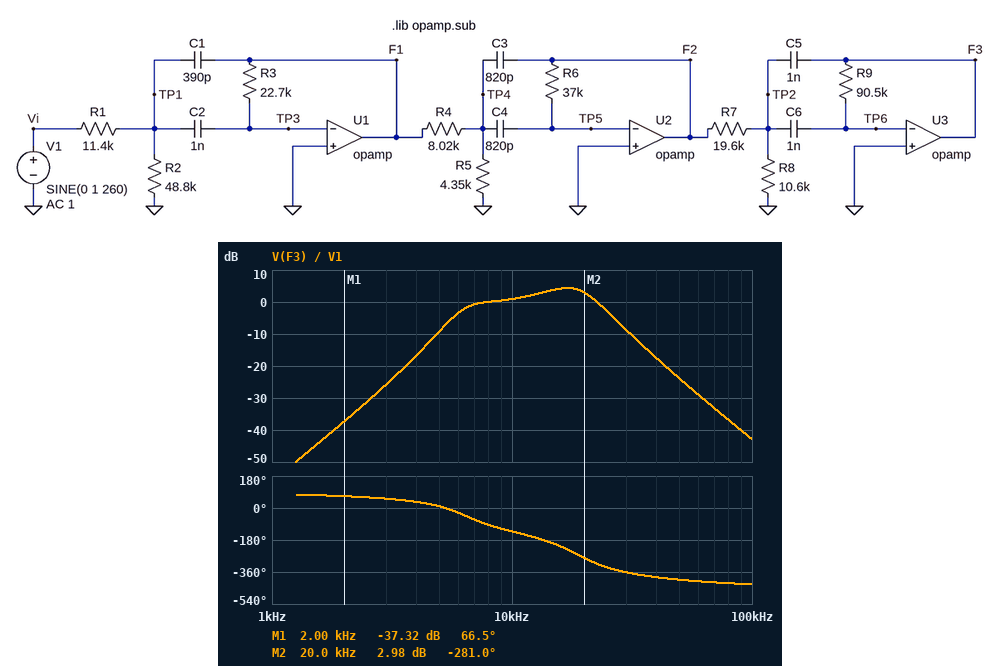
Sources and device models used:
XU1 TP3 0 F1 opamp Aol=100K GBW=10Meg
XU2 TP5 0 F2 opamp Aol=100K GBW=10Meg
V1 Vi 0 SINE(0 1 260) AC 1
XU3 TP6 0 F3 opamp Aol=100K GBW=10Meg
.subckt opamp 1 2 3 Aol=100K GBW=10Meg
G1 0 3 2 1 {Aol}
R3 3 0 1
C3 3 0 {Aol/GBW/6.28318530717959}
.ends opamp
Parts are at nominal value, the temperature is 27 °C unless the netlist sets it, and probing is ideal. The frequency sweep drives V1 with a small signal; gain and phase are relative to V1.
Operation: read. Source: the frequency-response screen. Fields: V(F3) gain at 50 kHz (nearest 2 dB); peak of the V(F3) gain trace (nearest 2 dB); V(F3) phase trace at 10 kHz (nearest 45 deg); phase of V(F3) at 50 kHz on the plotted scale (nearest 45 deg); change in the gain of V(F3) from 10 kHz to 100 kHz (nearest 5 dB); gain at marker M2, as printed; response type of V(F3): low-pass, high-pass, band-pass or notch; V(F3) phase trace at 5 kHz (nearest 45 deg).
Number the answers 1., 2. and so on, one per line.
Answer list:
1. -24 dB
2. 4 dB
3. -135 deg
4. -405 deg
5. -45 dB
6. 2.98 dB
7. band-pass
8. 0 deg
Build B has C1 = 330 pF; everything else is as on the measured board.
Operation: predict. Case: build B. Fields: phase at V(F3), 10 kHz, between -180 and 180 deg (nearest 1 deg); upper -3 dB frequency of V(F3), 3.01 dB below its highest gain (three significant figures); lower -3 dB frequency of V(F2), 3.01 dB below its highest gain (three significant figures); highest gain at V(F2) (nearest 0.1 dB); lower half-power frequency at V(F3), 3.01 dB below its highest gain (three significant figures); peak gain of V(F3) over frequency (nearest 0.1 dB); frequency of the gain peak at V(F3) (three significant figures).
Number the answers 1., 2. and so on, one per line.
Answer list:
1. -128 deg
2. 21.8 kHz
3. 14.9 kHz
4. 10.8 dB
5. 11.4 kHz
6. 4.7 dB
7. 17.3 kHz
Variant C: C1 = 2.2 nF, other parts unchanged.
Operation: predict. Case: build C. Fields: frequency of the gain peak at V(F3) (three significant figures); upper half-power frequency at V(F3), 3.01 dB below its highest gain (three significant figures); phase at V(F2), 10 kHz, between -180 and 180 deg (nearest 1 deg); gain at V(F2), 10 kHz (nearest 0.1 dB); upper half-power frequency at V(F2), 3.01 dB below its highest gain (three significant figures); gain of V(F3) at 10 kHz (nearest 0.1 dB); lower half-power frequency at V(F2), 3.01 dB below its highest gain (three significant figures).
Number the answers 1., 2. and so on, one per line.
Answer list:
1. 7.17 kHz
2. 12.0 kHz
3. 44 deg
4. -6.2 dB
5. 22.3 kHz
6. -4.8 dB
7. 11.6 kHz
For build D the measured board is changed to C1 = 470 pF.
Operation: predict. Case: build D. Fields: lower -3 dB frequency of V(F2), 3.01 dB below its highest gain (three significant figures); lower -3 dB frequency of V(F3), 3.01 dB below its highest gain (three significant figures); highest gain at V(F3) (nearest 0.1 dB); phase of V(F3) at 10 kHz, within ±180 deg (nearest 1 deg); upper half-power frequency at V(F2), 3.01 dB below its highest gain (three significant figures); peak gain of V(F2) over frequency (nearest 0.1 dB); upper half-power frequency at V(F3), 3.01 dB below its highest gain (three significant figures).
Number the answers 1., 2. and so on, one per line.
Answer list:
1. 14.3 kHz
2. 9.82 kHz
3. 3.9 dB
4. -136 deg
5. 23.4 kHz
6. 9.7 dB
7. 21.2 kHz
